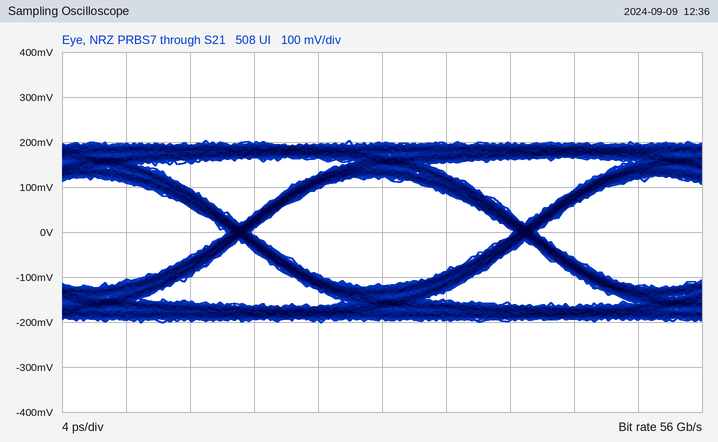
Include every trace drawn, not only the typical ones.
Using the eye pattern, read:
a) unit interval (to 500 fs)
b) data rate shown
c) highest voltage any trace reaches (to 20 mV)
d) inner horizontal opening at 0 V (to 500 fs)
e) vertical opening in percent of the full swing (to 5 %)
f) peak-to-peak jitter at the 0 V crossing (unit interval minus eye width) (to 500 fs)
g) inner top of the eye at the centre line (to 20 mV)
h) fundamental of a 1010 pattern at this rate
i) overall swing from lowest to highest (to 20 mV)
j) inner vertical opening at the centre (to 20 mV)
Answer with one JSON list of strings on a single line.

["18.0 ps", "56 Gb/s", "200 mV", "16.5 ps", "60 %", "1.5 ps", "120 mV", "28 GHz", "400 mV", "240 mV"]
